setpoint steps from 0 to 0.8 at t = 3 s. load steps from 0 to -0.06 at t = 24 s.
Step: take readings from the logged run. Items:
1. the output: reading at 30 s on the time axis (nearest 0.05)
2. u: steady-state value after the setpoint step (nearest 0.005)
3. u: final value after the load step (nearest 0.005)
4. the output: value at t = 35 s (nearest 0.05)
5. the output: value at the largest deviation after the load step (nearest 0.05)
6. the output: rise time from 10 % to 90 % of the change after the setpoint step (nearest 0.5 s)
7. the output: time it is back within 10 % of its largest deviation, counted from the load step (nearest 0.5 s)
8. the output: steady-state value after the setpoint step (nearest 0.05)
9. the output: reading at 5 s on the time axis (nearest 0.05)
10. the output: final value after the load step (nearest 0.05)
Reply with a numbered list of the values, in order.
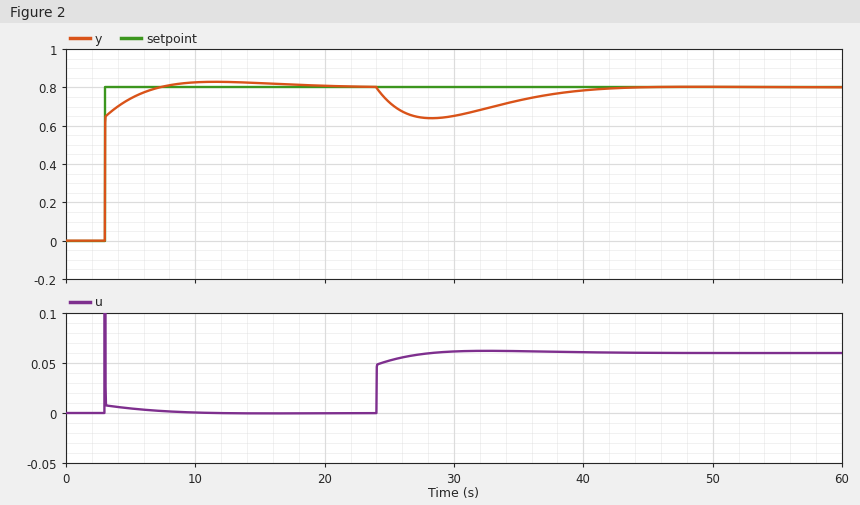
1. 0.65
2. 0.000
3. 0.060
4. 0.75
5. 0.65
6. 1.5 s
7. 16.0 s
8. 0.80
9. 0.75
10. 0.80
